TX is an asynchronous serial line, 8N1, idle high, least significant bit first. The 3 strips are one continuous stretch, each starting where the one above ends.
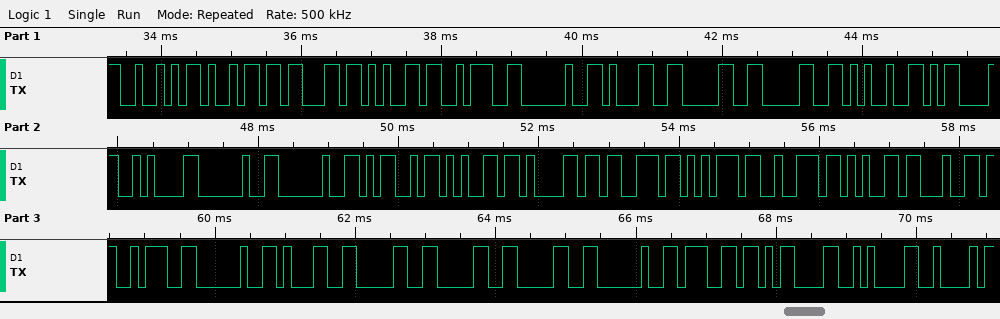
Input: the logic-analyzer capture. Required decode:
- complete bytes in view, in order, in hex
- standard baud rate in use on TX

52 69 63 65 3A 20 31 30 30 25 0D 0A 20 20 4D 65 61 73 75 72 65 64 3A 20 31 30 30 30 20 67 0D 0A 42
9600 baud
